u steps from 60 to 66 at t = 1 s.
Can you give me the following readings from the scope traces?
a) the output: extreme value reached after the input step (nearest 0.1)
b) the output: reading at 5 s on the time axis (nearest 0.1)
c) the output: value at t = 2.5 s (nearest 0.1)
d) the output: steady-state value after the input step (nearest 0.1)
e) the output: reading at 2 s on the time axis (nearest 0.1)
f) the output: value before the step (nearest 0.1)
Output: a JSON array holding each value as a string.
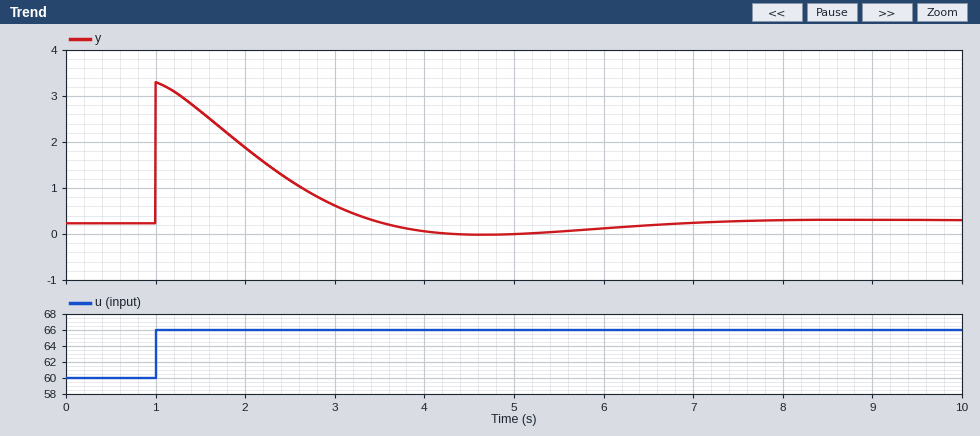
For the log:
["3.3", "0.0", "1.2", "0.3", "1.9", "0.2"]
